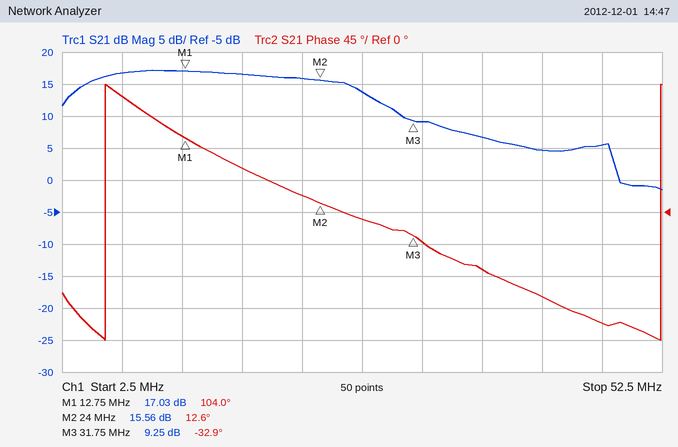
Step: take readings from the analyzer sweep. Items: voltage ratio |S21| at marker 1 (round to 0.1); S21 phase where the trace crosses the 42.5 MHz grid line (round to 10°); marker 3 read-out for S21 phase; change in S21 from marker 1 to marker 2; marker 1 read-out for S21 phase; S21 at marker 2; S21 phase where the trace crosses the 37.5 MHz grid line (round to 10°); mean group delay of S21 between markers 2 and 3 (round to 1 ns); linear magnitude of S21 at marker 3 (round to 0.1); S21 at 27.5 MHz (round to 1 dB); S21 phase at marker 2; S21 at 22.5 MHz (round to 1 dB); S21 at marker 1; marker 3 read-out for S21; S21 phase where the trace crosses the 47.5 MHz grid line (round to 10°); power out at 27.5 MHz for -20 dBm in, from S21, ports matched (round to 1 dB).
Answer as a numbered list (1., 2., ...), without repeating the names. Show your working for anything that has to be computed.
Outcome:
1. 10^(17.03/20) ≈ 7.1
2. -120°
3. -32.9°
4. 15.56 − (17.03) = -1.47 dB
5. 104.0°
6. 15.56 dB
7. -80°
8. −(-32.9° − (12.6°))/(360° × 7.75 MHz) ≈ 16 ns
9. 10^(9.25/20) ≈ 2.9
10. 14 dB
11. 12.6°
12. 16 dB
13. 17.03 dB
14. 9.25 dB
15. -160°
16. -20 dBm + (14 dB) = -6 dBm
